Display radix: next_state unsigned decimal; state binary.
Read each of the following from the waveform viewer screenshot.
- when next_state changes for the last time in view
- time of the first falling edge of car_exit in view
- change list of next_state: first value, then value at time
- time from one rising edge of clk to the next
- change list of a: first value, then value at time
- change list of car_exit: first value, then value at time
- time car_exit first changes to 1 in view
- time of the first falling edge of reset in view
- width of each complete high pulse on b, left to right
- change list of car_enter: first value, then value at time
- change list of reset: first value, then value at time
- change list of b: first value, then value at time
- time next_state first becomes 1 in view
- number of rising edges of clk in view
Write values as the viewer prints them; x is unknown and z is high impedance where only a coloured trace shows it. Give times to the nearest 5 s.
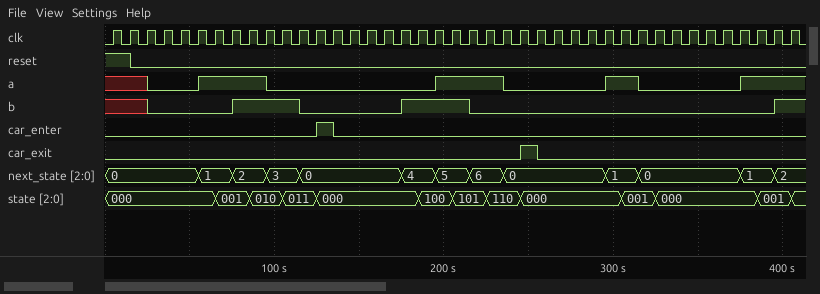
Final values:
395 s
255 s
0, 1 at 55 s, 2 at 75 s, 3 at 95 s, 0 at 115 s, 4 at 175 s, 5 at 195 s, 6 at 215 s, 0 at 235 s, 1 at 295 s, 0 at 315 s, 1 at 375 s, 2 at 395 s
10 s
x, 0 at 25 s, 1 at 55 s, 0 at 95 s, 1 at 195 s, 0 at 235 s, 1 at 295 s, 0 at 315 s, 1 at 375 s
0, 1 at 245 s, 0 at 255 s
245 s
15 s
40 s, 40 s
0, 1 at 125 s, 0 at 135 s
1, 0 at 15 s
x, 0 at 25 s, 1 at 75 s, 0 at 115 s, 1 at 175 s, 0 at 215 s, 1 at 395 s
55 s
41
